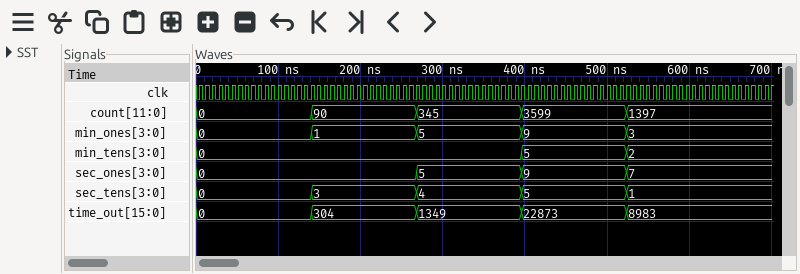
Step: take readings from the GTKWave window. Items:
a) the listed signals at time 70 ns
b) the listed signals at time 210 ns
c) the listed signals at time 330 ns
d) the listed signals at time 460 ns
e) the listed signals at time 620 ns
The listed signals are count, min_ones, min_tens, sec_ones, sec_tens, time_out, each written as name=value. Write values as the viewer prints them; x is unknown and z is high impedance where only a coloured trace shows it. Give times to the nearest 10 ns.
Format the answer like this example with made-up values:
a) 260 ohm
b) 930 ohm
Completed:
a) count=0, min_ones=0, min_tens=0, sec_ones=0, sec_tens=0, time_out=0
b) count=90, min_ones=1, min_tens=0, sec_ones=0, sec_tens=3, time_out=304
c) count=345, min_ones=5, min_tens=0, sec_ones=5, sec_tens=4, time_out=1349
d) count=3599, min_ones=9, min_tens=5, sec_ones=9, sec_tens=5, time_out=22873
e) count=1397, min_ones=3, min_tens=2, sec_ones=7, sec_tens=1, time_out=8983
